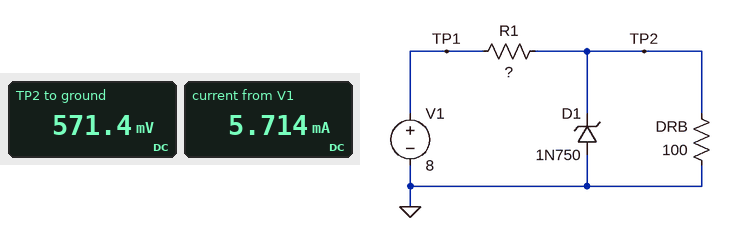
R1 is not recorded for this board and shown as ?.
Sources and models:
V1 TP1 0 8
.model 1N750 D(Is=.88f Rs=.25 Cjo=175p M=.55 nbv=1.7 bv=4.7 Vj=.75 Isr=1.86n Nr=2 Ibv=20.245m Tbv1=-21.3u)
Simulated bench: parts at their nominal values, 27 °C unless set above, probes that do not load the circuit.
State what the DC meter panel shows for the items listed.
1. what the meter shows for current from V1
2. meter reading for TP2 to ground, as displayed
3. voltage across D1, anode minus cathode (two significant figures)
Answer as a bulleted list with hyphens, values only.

- 5.714 mA
- 571.4 mV
- -570 mV
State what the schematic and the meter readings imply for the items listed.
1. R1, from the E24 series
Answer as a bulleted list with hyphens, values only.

- 1.3 kΩ
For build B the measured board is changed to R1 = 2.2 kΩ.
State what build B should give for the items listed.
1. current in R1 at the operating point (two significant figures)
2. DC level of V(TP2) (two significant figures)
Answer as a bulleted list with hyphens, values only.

- 3.5 mA
- 350 mV
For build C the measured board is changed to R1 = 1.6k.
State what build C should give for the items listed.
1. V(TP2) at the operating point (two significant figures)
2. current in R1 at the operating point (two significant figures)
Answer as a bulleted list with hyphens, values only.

- 470 mV
- 4.7 mA
